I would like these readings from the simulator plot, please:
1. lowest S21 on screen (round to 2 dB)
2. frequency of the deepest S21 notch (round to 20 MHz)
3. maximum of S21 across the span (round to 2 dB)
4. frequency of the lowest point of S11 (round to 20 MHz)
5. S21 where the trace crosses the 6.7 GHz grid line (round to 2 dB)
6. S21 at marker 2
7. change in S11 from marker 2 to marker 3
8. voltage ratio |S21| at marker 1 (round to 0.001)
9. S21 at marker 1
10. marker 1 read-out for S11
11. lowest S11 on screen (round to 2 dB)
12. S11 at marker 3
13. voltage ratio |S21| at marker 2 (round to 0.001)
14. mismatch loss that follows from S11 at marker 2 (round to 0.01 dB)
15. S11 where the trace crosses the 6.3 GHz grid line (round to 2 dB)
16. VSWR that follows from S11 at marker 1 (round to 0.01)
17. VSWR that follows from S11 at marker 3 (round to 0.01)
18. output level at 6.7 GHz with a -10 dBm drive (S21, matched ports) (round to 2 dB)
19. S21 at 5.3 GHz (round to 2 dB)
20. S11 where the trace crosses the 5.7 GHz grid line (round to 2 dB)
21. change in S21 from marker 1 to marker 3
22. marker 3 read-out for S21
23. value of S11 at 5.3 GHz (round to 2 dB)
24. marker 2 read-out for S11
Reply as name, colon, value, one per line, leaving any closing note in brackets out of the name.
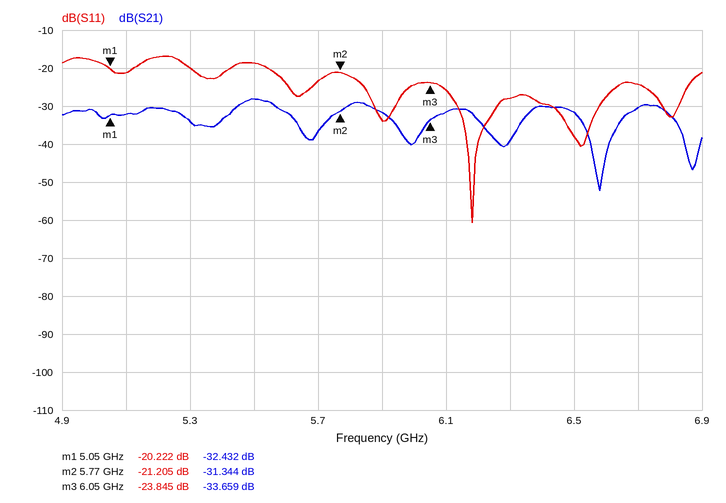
lowest S21 on screen: -52 dB
frequency of the deepest S21 notch: 6.58 GHz
maximum of S21 across the span: -28 dB
frequency of the lowest point of S11: 6.18 GHz
S21 where the trace crosses the 6.7 GHz grid line: -30 dB
S21 at marker 2: -31.344 dB
change in S11 from marker 2 to marker 3: -2.640 dB
voltage ratio |S21| at marker 1: 0.024
S21 at marker 1: -32.432 dB
marker 1 read-out for S11: -20.222 dB
lowest S11 on screen: -60 dB
S11 at marker 3: -23.845 dB
voltage ratio |S21| at marker 2: 0.027
mismatch loss that follows from S11 at marker 2: 0.03 dB
S11 where the trace crosses the 6.3 GHz grid line: -28 dB
VSWR that follows from S11 at marker 1: 1.22
VSWR that follows from S11 at marker 3: 1.14
output level at 6.7 GHz with a -10 dBm drive (S21, matched ports): -40 dBm
S21 at 5.3 GHz: -34 dB
S11 where the trace crosses the 5.7 GHz grid line: -24 dB
change in S21 from marker 1 to marker 3: -1.227 dB
marker 3 read-out for S21: -33.659 dB
value of S11 at 5.3 GHz: -20 dB
marker 2 read-out for S11: -21.205 dB
